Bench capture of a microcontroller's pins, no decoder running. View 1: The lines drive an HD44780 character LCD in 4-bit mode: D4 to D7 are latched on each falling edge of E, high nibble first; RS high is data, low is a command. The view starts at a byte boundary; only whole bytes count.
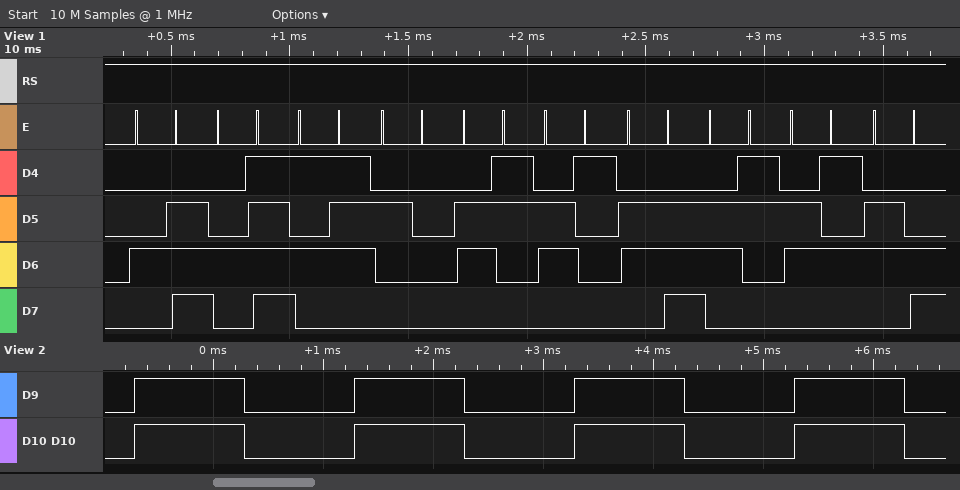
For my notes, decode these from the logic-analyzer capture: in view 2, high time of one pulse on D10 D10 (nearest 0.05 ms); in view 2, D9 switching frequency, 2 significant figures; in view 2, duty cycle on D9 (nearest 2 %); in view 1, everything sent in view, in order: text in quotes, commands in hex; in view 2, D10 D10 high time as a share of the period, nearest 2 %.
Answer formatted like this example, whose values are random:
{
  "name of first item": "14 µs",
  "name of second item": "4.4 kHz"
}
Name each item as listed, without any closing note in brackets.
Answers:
{
  "in view 2, high time of one pulse on D10 D10": "1.00 ms",
  "in view 2, D9 switching frequency, 2 significant figures": "500 Hz",
  "in view 2, duty cycle on D9": "50 %",
  "in view 1, everything sent in view, in order: text in quotes, commands in hex": "\"NOW cancel\"",
  "in view 2, D10 D10 high time as a share of the period, nearest 2 %": "50 %"
}
